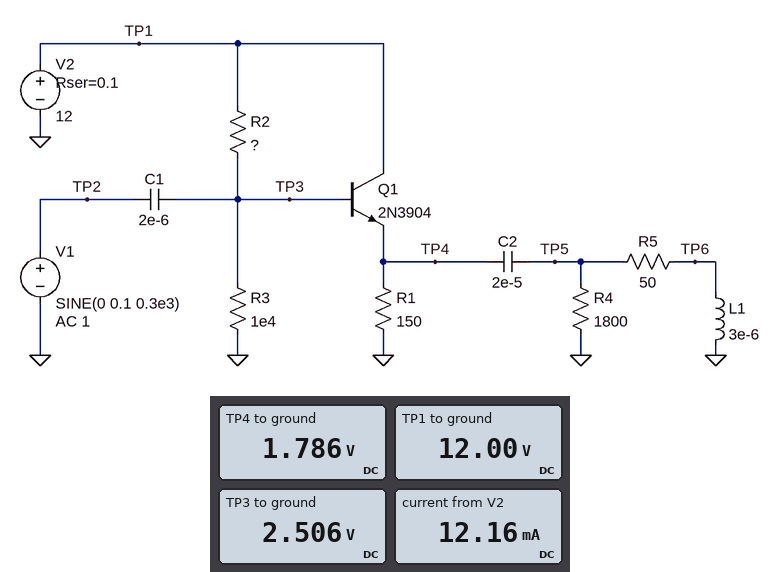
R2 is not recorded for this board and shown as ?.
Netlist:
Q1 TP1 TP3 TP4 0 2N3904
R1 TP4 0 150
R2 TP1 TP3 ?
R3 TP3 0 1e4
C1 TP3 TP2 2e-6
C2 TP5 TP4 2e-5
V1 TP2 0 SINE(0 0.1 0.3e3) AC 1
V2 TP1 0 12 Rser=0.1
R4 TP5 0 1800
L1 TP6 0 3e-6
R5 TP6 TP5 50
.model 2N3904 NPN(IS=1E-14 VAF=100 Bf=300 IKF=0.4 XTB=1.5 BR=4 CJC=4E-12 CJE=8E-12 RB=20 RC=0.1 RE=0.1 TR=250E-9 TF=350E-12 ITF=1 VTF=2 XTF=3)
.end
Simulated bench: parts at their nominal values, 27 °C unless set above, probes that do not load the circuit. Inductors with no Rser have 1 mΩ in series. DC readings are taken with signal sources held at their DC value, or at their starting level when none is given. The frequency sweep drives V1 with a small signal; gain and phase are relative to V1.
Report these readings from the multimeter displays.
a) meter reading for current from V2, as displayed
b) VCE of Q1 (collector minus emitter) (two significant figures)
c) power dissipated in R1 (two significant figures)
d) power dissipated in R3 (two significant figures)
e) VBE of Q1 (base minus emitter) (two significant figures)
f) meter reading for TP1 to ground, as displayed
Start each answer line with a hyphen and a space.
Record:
- 12.16 mA
- 10 V
- 21 mW
- 630 µW
- 720 mV
- 12.00 V
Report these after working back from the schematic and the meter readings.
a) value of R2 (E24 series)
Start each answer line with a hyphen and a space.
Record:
- 33 kΩ
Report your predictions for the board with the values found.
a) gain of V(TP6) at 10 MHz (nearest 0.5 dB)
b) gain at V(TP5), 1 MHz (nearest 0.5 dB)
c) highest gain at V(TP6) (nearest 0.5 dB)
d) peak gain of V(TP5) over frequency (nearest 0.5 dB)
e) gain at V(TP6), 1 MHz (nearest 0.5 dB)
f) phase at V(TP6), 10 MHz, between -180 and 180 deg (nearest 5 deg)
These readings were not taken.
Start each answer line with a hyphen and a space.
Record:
- -0.5 dB
- -0.5 dB
- 0 dB
- 0 dB
- -9.5 dB
- 15 deg
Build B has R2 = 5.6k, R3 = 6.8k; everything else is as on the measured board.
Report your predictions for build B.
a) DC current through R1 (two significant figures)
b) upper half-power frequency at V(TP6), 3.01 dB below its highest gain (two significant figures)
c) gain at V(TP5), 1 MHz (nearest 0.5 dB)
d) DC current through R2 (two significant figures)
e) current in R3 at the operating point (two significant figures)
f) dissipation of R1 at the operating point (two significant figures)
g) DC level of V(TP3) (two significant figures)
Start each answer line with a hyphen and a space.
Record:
- 36 mA
- 3.4 GHz
- 0 dB
- 1.0 mA
- 910 µA
- 200 mW
- 6.2 V
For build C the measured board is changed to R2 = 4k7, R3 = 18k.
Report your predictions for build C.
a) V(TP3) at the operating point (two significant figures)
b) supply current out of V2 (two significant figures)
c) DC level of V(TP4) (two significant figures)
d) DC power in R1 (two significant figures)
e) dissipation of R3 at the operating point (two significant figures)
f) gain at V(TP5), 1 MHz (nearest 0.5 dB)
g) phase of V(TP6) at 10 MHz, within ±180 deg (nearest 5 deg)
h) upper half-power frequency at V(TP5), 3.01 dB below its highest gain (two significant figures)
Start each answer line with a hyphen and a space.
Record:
- 8.8 V
- 54 mA
- 8.0 V
- 430 mW
- 4.3 mW
- 0 dB
- 15 deg
- 2.8 GHz
